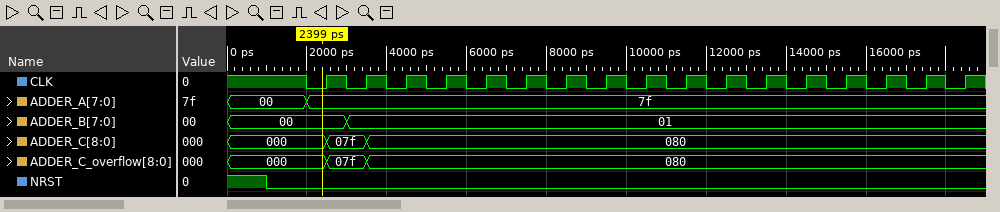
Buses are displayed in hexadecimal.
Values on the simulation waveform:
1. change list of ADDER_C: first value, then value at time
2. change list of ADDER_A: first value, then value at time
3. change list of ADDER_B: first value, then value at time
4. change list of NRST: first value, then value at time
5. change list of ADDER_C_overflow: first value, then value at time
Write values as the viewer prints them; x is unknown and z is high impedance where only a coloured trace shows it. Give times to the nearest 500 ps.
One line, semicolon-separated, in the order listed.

000, 07f at 2500 ps, 080 at 3500 ps; 00, 7f at 2000 ps; 00, 01 at 3000 ps; 1, 0 at 1000 ps; 000, 07f at 2500 ps, 080 at 3500 ps
